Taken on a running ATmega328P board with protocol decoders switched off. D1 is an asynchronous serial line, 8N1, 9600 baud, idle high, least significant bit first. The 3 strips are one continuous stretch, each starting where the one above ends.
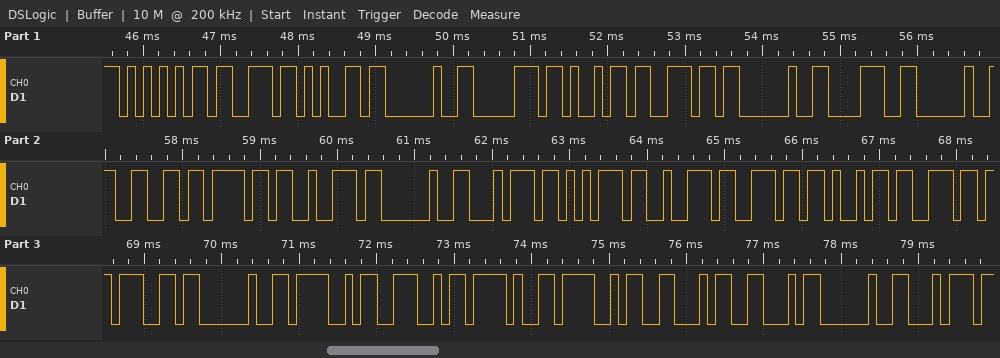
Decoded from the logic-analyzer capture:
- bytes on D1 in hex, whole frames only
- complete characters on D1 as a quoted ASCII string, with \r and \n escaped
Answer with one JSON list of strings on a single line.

["55 73 65 20 70 69 6E 20 38 20 66 6F 72 20 74 75 72 6E 69 6E 67 20 4F 4E 2F 4F 46 46 20 74", "\"Use pin 8 for turning ON/OFF t\""]
